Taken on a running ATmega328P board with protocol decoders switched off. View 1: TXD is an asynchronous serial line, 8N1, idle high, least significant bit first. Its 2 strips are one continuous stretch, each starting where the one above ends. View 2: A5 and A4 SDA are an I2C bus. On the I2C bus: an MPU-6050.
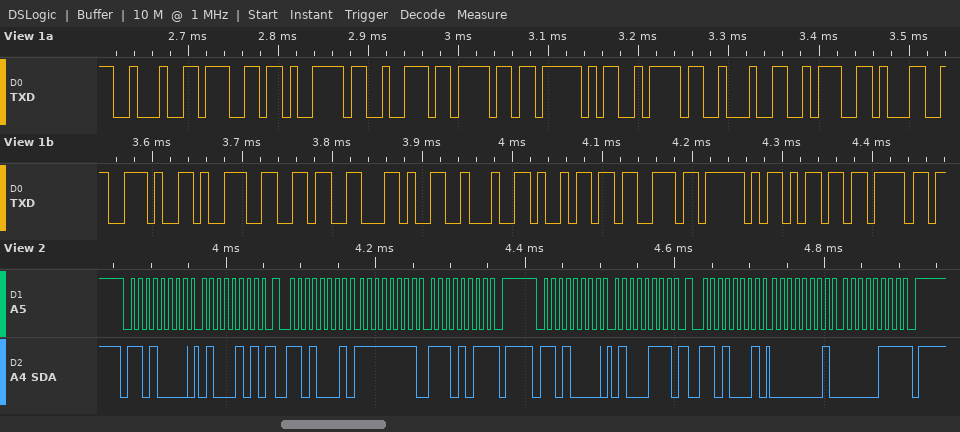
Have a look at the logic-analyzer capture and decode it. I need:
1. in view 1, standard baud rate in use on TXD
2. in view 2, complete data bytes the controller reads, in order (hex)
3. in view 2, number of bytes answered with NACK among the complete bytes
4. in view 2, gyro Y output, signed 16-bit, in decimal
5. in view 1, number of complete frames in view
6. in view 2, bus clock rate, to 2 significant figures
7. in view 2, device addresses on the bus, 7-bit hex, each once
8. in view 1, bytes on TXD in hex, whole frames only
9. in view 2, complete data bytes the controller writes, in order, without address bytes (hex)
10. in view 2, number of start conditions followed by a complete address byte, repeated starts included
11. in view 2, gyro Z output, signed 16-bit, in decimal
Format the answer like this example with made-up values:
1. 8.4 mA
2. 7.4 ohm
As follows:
1. 115200 baud
2. FF EB 01 07
3. 2
4. -21
5. 20
6. 100 kHz
7. 0x68
8. 0x22 0x67 0x79 0x72 0x6F 0x5F 0x7A 0x22 0x3A 0x31 0x2E 0x39 0x36 0x2C 0x22 0x69 0x73 0x5F 0x6D 0x6F
9. 45 47
10. 4
11. 263
